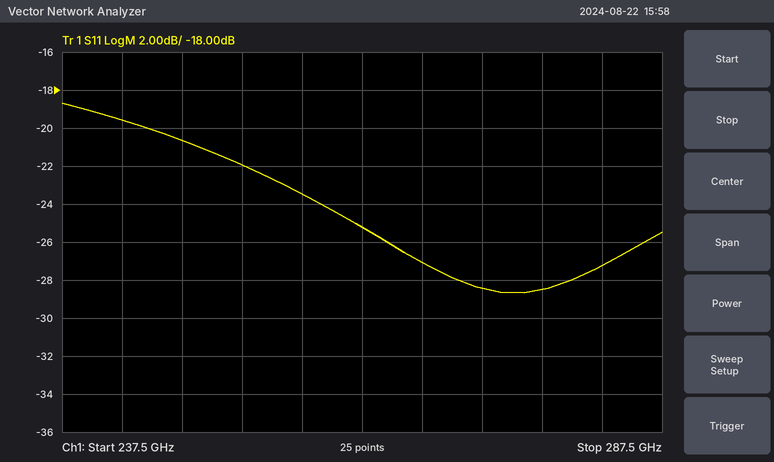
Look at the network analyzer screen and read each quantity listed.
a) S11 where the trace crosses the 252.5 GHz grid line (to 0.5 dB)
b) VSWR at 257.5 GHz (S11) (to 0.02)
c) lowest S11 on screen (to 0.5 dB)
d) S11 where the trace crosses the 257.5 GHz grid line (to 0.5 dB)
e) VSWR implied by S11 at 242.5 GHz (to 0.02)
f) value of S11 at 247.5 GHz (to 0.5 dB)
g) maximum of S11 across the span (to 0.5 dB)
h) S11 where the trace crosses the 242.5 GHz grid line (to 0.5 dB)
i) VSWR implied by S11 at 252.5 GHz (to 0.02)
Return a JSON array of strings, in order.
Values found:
["-22.0 dB", "1.14", "-28.5 dB", "-23.5 dB", "1.24", "-20.5 dB", "-18.5 dB", "-19.5 dB", "1.18"]
